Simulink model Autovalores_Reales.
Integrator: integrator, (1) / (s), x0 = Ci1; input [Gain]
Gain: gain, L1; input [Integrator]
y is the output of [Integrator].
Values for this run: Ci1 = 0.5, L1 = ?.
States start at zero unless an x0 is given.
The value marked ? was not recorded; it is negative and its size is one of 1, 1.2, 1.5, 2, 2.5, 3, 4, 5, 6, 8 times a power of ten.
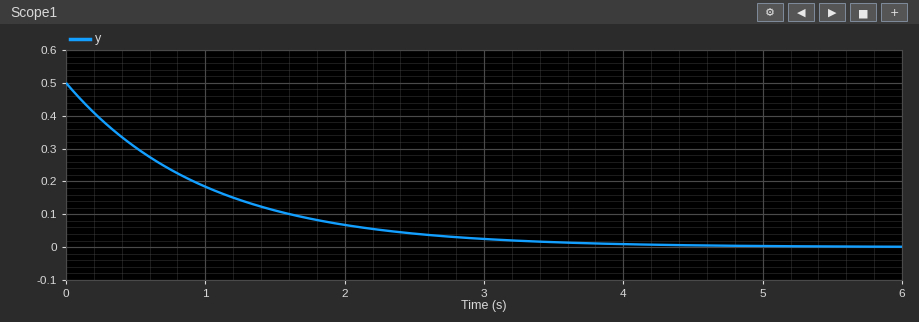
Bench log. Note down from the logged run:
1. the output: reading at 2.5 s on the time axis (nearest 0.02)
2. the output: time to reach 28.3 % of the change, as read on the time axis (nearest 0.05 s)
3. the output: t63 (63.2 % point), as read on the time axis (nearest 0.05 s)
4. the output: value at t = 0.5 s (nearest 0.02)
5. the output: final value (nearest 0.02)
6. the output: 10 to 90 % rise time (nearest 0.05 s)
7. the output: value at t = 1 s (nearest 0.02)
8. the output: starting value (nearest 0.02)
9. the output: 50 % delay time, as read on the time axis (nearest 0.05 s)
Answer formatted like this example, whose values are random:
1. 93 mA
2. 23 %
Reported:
1. 0.04
2. 0.35 s
3. 1.00 s
4. 0.30
5. 0.00
6. 2.20 s
7. 0.18
8. 0.50
9. 0.70 s
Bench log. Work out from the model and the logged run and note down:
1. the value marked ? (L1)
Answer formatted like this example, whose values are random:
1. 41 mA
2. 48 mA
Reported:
1. -1
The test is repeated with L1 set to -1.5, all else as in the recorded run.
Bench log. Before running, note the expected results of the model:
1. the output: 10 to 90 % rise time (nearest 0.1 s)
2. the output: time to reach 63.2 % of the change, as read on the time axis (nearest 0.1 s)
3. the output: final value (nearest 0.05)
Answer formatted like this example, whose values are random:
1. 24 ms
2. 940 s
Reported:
1. 1.5 s
2. 0.7 s
3. 0.00
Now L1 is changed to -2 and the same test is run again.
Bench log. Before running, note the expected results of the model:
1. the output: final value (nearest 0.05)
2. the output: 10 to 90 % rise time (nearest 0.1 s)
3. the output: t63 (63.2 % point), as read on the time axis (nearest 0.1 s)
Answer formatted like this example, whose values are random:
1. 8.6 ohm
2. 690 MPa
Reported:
1. 0.00
2. 1.1 s
3. 0.5 s
